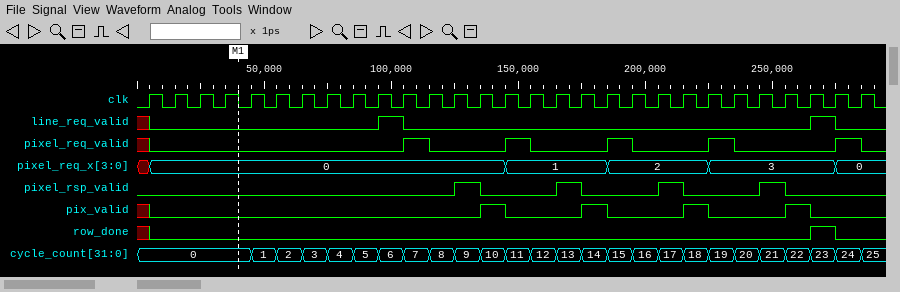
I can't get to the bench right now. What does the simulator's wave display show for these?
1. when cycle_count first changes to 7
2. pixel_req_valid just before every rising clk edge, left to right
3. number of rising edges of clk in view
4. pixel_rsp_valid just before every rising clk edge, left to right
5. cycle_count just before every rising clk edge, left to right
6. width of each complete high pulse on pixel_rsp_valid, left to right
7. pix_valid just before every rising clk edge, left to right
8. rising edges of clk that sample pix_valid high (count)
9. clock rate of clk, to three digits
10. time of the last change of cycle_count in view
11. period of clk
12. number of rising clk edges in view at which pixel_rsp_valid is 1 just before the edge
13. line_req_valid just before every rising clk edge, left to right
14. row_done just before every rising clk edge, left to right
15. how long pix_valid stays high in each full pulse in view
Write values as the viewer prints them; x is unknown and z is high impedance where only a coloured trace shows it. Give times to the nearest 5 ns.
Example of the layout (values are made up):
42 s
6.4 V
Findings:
105 ns
x 0 0 0 0 0 0 0 0 0 0 1 0 0 0 1 0 0 0 1 0 0 0 1 0 0 0 0 1
29
0 0 0 0 0 0 0 0 0 0 0 0 0 1 0 0 0 1 0 0 0 1 0 0 0 1 0 0 0
0, 0, 0, 0, 0, 1, 2, 3, 4, 5, 6, 7, 8, 9, 10, 11, 12, 13, 14, 15, 16, 17, 18, 19, 20, 21, 22, 23, 24
10 ns, 10 ns, 10 ns, 10 ns
x 0 0 0 0 0 0 0 0 0 0 0 0 0 1 0 0 0 1 0 0 0 1 0 0 0 1 0 0
4
100 MHz
285 ns
10 ns
4
x 0 0 0 0 0 0 0 0 0 1 0 0 0 0 0 0 0 0 0 0 0 0 0 0 0 0 1 0
x 0 0 0 0 0 0 0 0 0 0 0 0 0 0 0 0 0 0 0 0 0 0 0 0 0 0 1 0
10 ns, 10 ns, 10 ns, 10 ns
